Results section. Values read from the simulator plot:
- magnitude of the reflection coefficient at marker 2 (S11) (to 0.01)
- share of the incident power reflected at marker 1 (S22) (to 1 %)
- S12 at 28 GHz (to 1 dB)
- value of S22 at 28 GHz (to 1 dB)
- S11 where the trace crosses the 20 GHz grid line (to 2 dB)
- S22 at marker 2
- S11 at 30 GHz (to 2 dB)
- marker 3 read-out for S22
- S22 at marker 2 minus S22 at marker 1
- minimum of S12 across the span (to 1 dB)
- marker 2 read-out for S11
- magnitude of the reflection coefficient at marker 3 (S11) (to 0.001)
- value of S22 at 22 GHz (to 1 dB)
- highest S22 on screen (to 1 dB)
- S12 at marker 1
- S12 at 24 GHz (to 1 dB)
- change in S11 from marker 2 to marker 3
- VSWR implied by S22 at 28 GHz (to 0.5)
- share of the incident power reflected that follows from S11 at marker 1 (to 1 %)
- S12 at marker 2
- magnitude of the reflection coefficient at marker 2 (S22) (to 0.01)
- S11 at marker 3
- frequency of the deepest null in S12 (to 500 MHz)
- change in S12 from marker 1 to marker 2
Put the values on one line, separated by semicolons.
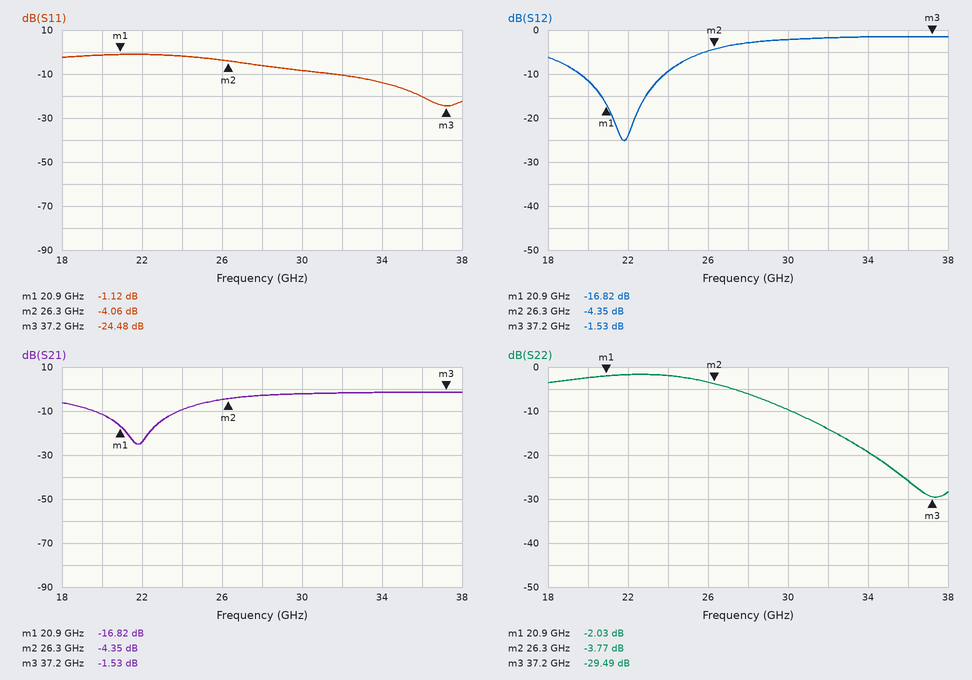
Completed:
0.63; 63 %; -3 dB; -6 dB; -2 dB; -3.77 dB; -8 dB; -29.49 dB; -1.74 dB; -25 dB; -4.06 dB; 0.060; -2 dB; -2 dB; -16.82 dB; -9 dB; -20.42 dB; 3.0; 77 %; -4.35 dB; 0.65; -24.48 dB; 22.0 GHz; 12.47 dB
